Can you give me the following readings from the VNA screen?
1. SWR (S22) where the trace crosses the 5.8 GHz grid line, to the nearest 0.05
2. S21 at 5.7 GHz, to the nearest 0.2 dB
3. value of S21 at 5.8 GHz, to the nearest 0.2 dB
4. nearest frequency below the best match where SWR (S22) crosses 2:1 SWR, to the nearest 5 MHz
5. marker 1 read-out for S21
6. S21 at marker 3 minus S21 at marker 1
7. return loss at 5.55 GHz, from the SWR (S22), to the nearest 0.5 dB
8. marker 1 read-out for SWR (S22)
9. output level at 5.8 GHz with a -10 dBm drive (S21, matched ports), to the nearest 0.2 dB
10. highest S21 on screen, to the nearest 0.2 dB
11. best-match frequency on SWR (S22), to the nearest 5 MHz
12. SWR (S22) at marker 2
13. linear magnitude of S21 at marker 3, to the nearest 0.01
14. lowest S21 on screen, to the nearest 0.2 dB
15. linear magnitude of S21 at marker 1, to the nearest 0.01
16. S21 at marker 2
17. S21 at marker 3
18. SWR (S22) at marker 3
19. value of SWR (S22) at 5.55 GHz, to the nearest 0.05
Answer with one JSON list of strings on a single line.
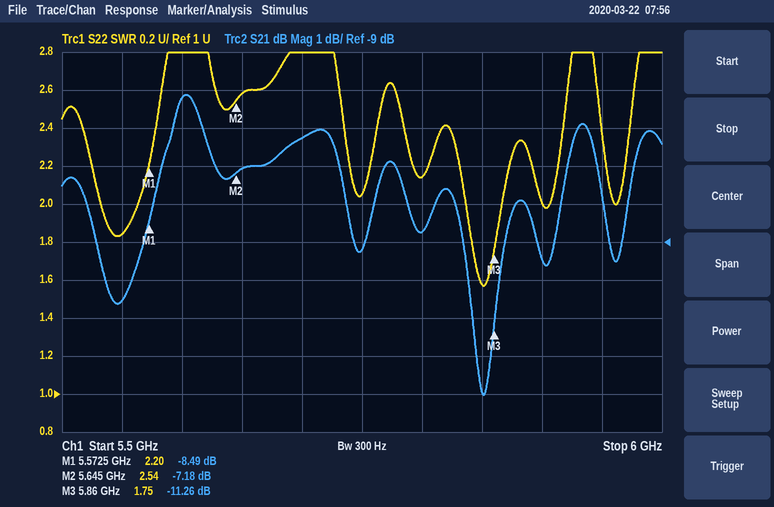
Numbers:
["2.15", "-6.2 dB", "-8.8 dB", "5.835 GHz", "-8.49 dB", "-2.77 dB", "10.5 dB", "2.20", "-18.8 dBm", "-5.2 dB", "5.850 GHz", "2.54", "0.27", "-13.0 dB", "0.38", "-7.18 dB", "-11.26 dB", "1.75", "1.85"]
